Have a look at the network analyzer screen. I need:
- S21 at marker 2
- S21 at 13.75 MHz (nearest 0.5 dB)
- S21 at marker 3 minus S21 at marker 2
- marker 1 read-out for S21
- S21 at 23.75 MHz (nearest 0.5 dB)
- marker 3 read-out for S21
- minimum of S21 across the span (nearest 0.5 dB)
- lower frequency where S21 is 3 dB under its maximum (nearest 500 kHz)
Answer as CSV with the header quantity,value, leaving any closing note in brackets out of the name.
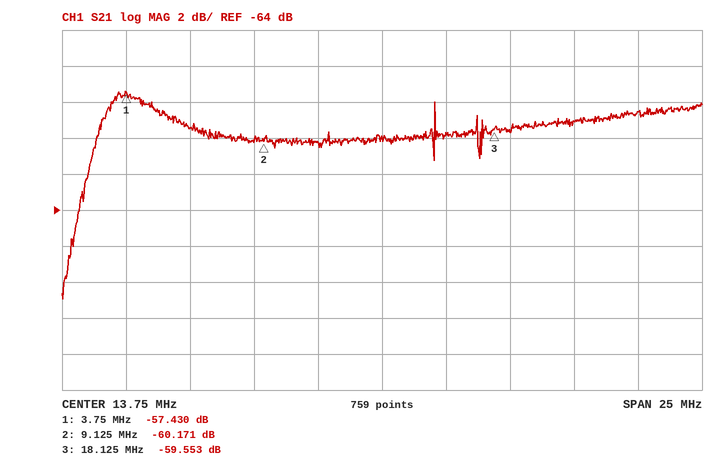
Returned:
quantity,value
S21 at marker 2,-60.171 dB
S21 at 13.75 MHz,-60.0 dB
S21 at marker 3 minus S21 at marker 2,0.618 dB
marker 1 read-out for S21,-57.430 dB
S21 at 23.75 MHz,-58.5 dB
marker 3 read-out for S21,-59.553 dB
minimum of S21 across the span,-69.0 dB
lower frequency where S21 is 3 dB under its maximum,2.5 MHz
